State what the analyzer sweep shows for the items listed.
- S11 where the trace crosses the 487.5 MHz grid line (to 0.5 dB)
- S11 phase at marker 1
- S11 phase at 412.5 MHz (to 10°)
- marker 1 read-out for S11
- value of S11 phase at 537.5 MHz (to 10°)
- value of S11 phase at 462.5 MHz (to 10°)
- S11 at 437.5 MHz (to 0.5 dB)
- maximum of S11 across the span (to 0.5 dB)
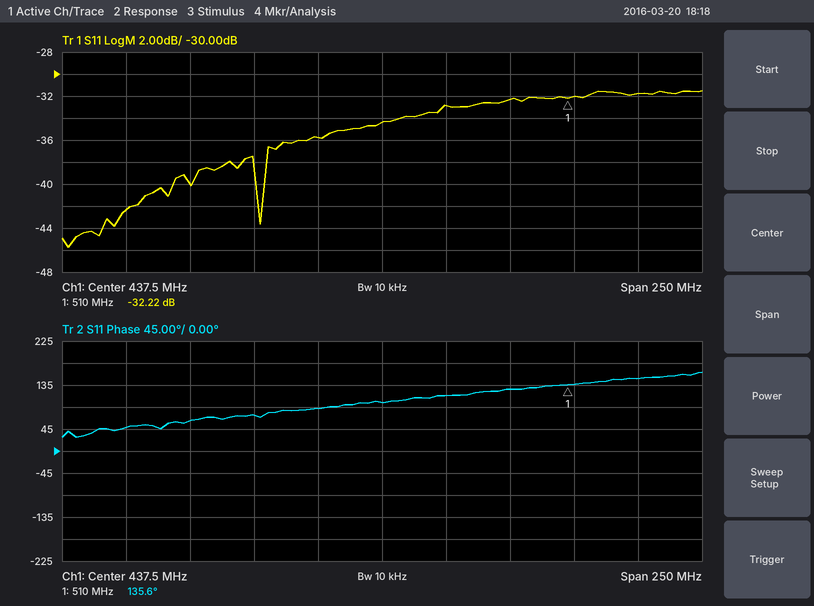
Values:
-32.5 dB
135.6°
90°
-32.22 dB
150°
110°
-34.5 dB
-31.5 dB
